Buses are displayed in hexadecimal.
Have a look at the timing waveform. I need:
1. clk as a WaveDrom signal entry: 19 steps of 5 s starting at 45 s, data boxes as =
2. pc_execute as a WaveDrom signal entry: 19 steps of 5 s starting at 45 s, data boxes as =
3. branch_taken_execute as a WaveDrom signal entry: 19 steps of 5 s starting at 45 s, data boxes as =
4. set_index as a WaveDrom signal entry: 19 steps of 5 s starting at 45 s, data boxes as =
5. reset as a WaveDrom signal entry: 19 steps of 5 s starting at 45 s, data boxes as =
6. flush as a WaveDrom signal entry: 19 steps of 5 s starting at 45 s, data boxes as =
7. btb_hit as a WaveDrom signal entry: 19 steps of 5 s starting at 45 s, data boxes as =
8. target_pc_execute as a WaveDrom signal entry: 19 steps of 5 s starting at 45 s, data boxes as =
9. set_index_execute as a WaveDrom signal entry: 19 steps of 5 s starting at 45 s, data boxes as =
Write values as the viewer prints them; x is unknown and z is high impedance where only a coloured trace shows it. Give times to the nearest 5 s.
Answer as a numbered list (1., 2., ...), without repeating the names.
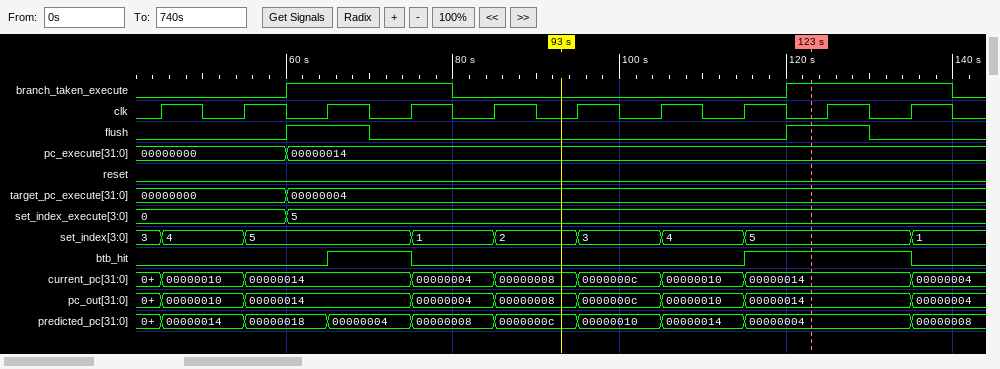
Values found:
1. {name: 'clk', wave: '1010101010101010101'}
2. {name: 'pc_execute', wave: '=..=...............', data: '00000000 00000014'}
3. {name: 'branch_taken_execute', wave: '0..1...0.......1...'}
4. {name: 'set_index', wave: '=.=...=.=.=.=.=...=', data: '4 5 1 2 3 4 5 1'}
5. {name: 'reset', wave: '0..................'}
6. {name: 'flush', wave: '0..1.0.........1.0.'}
7. {name: 'btb_hit', wave: '0...1.0.......1...0'}
8. {name: 'target_pc_execute', wave: '=..=...............', data: '00000000 00000004'}
9. {name: 'set_index_execute', wave: '=..=...............', data: '0 5'}
